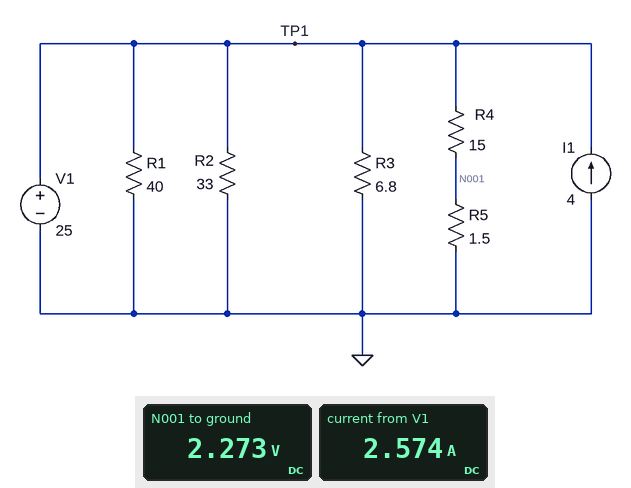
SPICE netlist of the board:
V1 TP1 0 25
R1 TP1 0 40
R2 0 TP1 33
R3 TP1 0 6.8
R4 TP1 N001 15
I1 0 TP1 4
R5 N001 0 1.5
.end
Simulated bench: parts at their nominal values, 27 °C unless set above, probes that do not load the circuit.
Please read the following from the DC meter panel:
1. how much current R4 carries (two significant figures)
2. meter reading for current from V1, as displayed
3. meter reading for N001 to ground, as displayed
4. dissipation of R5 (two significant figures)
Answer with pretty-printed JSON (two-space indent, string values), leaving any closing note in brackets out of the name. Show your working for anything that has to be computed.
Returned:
{
  "how much current R4 carries": "(25 V - 2.273 V) / 15 Ω = 1.5 A",
  "meter reading for current from V1, as displayed": "2.574 A",
  "meter reading for N001 to ground, as displayed": "2.273 V",
  "dissipation of R5": "(2.273 V)^2 / 1.5 Ω = 3.4 W"
}
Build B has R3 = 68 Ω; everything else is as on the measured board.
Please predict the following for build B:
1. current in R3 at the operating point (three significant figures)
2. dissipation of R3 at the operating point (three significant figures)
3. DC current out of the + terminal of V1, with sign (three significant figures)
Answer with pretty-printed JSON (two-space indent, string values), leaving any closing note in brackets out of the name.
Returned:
{
  "current in R3 at the operating point": "368 mA",
  "dissipation of R3 at the operating point": "9.19 W",
  "DC current out of the + terminal of V1, with sign": "-735 mA"
}
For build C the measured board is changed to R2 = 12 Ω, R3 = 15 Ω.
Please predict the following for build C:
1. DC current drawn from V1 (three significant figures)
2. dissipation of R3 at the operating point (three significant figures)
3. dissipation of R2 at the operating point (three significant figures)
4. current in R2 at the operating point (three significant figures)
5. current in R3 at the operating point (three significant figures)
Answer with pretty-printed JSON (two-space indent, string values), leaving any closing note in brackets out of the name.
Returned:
{
  "DC current drawn from V1": "1.89 A",
  "dissipation of R3 at the operating point": "41.7 W",
  "dissipation of R2 at the operating point": "52.1 W",
  "current in R2 at the operating point": "2.08 A",
  "current in R3 at the operating point": "1.67 A"
}
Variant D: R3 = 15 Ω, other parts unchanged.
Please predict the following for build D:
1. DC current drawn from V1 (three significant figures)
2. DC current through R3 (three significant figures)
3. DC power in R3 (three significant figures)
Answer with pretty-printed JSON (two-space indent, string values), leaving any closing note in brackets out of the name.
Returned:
{
  "DC current drawn from V1": "564 mA",
  "DC current through R3": "1.67 A",
  "DC power in R3": "41.7 W"
}
